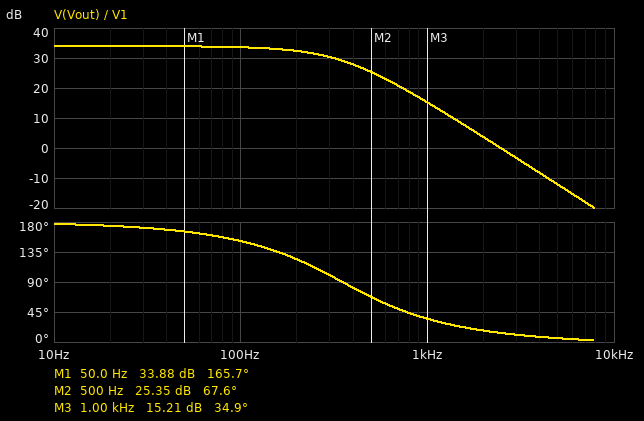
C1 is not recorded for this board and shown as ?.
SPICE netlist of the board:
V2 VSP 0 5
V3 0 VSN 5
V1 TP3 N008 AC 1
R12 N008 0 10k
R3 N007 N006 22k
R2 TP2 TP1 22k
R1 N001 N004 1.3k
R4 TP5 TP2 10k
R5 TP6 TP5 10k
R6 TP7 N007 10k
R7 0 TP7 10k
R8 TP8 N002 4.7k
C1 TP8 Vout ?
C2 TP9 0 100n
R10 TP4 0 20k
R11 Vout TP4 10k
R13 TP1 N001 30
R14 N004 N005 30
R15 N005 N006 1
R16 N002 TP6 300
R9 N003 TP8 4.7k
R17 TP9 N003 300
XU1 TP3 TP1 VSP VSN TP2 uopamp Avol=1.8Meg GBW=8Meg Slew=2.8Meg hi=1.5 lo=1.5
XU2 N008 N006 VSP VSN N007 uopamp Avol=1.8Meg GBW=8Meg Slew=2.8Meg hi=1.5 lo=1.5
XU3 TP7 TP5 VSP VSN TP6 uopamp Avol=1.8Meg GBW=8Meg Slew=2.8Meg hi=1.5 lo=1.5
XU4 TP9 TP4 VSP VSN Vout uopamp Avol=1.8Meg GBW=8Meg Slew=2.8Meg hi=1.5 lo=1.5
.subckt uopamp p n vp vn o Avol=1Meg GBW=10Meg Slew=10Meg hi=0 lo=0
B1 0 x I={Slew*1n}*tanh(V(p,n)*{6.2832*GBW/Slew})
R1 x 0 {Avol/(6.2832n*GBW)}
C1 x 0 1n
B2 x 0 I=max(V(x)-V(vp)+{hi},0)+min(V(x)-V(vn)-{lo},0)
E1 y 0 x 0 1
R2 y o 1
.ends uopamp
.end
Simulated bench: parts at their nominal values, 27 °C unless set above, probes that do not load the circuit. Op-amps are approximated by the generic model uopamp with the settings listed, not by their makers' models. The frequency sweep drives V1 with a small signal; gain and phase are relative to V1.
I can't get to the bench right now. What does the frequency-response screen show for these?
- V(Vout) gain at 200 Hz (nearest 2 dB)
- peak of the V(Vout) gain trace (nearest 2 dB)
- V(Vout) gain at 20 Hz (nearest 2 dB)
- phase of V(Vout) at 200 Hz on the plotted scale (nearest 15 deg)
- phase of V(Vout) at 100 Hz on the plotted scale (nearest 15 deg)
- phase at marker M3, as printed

32 dB
34 dB
34 dB
120 deg
150 deg
34.9 deg
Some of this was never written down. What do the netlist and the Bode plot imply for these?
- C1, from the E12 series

82 nF
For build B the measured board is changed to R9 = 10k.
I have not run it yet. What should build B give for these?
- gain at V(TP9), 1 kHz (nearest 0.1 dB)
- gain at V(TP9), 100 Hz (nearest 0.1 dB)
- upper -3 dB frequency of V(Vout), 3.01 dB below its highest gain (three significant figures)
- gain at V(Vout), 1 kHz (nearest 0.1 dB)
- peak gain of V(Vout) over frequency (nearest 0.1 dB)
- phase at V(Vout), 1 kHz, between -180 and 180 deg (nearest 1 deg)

5.5 dB
29.0 dB
153 Hz
9.0 dB
34.0 dB
28 deg
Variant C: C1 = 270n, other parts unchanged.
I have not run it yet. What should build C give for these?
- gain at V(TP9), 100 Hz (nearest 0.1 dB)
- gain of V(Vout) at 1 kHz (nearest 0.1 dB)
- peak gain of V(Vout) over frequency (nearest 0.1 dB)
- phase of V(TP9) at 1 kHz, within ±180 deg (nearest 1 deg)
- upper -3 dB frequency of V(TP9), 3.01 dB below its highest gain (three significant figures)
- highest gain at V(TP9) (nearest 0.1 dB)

32.8 dB
5.8 dB
42.2 dB
4 deg
222 Hz
38.7 dB
